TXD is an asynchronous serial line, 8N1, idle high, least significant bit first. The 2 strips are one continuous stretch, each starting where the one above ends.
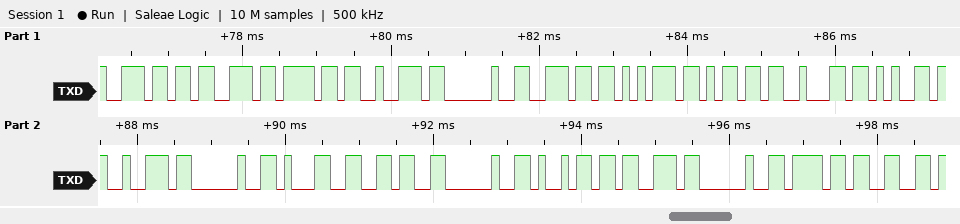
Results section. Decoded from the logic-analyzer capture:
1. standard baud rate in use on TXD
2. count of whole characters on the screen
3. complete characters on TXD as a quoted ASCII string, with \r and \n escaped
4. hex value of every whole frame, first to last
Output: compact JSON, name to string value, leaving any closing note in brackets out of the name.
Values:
{"standard baud rate in use on TXD": "9600 baud", "count of whole characters on the screen": "20", "complete characters on TXD as a quoted ASCII string, with \\r and \\n escaped": "\"nsor number 16 is of\"", "hex value of every whole frame, first to last": "6E 73 6F 72 20 6E 75 6D 62 65 72 20 31 36 20 69 73 20 6F 66"}
